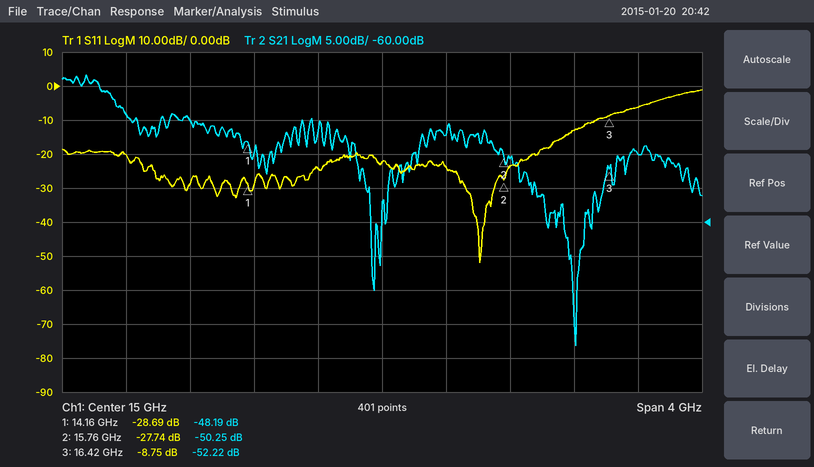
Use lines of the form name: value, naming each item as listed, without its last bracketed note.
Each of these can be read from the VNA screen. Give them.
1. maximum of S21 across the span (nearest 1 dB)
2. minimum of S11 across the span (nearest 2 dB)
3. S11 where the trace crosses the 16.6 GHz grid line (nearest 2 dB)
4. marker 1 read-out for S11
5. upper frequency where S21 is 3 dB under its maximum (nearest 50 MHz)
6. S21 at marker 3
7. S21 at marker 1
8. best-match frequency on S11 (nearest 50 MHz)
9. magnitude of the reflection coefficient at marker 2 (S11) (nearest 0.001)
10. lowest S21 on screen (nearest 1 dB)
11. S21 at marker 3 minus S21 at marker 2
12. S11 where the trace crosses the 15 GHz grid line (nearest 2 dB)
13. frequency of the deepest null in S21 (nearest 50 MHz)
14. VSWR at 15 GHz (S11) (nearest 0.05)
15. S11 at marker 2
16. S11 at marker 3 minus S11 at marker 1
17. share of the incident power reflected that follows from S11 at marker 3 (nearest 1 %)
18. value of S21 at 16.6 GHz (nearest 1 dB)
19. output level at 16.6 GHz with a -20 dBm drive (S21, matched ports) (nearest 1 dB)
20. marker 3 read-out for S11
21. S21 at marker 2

maximum of S21 across the span: -38 dB
minimum of S11 across the span: -52 dB
S11 where the trace crosses the 16.6 GHz grid line: -6 dB
marker 1 read-out for S11: -28.69 dB
upper frequency where S21 is 3 dB under its maximum: 13.30 GHz
S21 at marker 3: -52.22 dB
S21 at marker 1: -48.19 dB
best-match frequency on S11: 15.60 GHz
magnitude of the reflection coefficient at marker 2 (S11): 0.041
lowest S21 on screen: -78 dB
S21 at marker 3 minus S21 at marker 2: -1.97 dB
S11 where the trace crosses the 15 GHz grid line: -22 dB
frequency of the deepest null in S21: 16.20 GHz
VSWR at 15 GHz (S11): 1.15
S11 at marker 2: -27.74 dB
S11 at marker 3 minus S11 at marker 1: 19.94 dB
share of the incident power reflected that follows from S11 at marker 3: 13 %
value of S21 at 16.6 GHz: -50 dB
output level at 16.6 GHz with a -20 dBm drive (S21, matched ports): -70 dBm
marker 3 read-out for S11: -8.75 dB
S21 at marker 2: -50.25 dB
